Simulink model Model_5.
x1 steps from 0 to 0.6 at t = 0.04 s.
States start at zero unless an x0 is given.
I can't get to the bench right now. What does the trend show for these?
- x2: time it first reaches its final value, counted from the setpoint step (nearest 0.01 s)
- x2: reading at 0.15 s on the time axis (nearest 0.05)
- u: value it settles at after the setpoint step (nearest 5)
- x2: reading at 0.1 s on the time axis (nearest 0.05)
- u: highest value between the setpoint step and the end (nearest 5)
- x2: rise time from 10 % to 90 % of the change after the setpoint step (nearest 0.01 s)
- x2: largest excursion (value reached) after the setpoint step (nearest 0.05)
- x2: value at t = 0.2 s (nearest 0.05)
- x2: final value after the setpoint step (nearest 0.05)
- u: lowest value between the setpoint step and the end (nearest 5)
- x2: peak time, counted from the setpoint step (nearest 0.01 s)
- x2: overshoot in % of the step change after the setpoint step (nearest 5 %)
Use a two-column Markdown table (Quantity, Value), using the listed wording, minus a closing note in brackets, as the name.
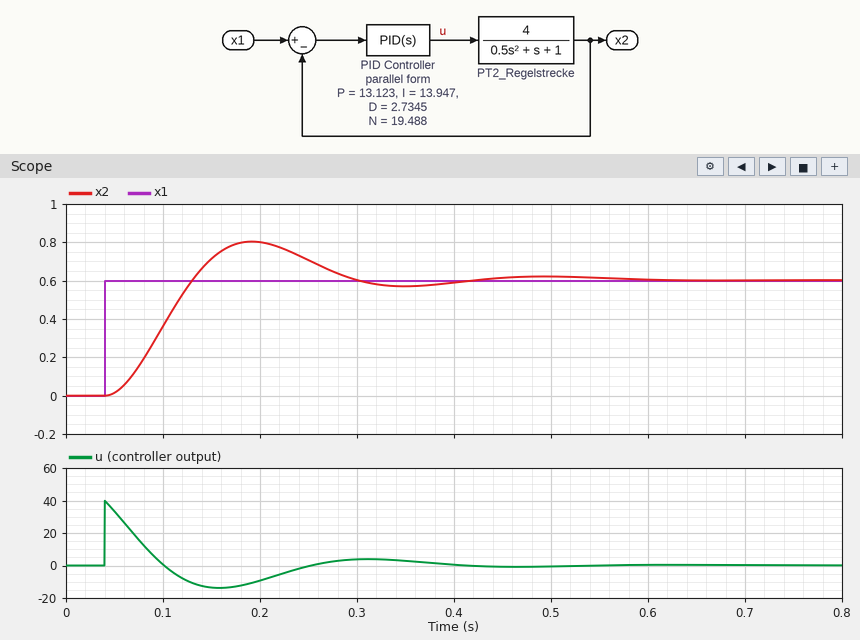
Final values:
| Quantity | Value |
|---|---|
| x2: time it first reaches its final value, counted from the setpoint step | 0.09 s |
| x2: reading at 0.15 s on the time axis | 0.70 |
| u: value it settles at after the setpoint step | 0 |
| x2: reading at 0.1 s on the time axis | 0.35 |
| u: highest value between the setpoint step and the end | 40 |
| x2: rise time from 10 % to 90 % of the change after the setpoint step | 0.06 s |
| x2: largest excursion (value reached) after the setpoint step | 0.80 |
| x2: value at t = 0.2 s | 0.80 |
| x2: final value after the setpoint step | 0.60 |
| u: lowest value between the setpoint step and the end | -15 |
| x2: peak time, counted from the setpoint step | 0.15 s |
| x2: overshoot in % of the step change after the setpoint step | 35 % |
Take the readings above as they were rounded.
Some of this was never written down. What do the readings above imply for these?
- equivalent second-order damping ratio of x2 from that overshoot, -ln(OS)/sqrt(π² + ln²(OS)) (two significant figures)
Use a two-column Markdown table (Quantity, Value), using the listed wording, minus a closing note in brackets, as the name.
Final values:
| Quantity | Value |
|---|---|
| equivalent second-order damping ratio of x2 from that overshoot, -ln(OS)/sqrt(π² + ln²(OS)) | 0.32 |
